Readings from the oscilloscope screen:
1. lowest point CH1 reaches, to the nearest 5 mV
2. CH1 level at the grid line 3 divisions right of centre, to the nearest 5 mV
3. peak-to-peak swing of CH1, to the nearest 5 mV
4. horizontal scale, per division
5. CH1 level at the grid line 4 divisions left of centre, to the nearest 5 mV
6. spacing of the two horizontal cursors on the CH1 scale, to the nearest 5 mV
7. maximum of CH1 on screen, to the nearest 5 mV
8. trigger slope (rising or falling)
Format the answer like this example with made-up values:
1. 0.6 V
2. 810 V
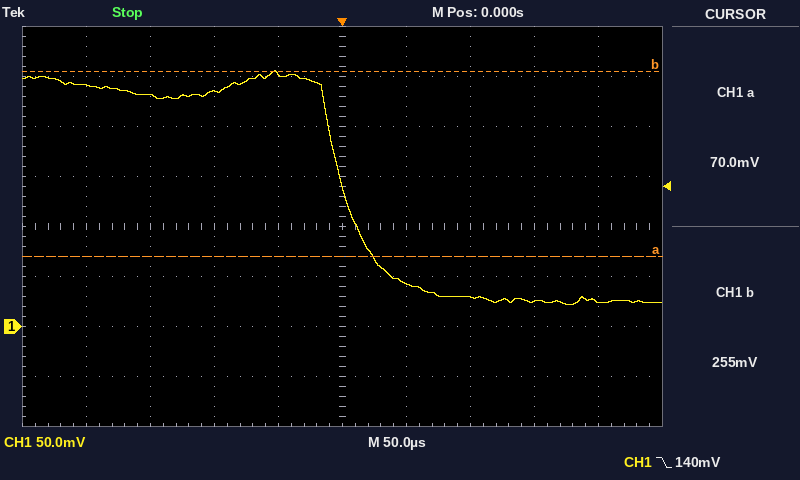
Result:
1. 20 mV
2. 25 mV
3. 235 mV
4. 50 µs
5. 240 mV
6. 185 mV
7. 255 mV
8. falling
